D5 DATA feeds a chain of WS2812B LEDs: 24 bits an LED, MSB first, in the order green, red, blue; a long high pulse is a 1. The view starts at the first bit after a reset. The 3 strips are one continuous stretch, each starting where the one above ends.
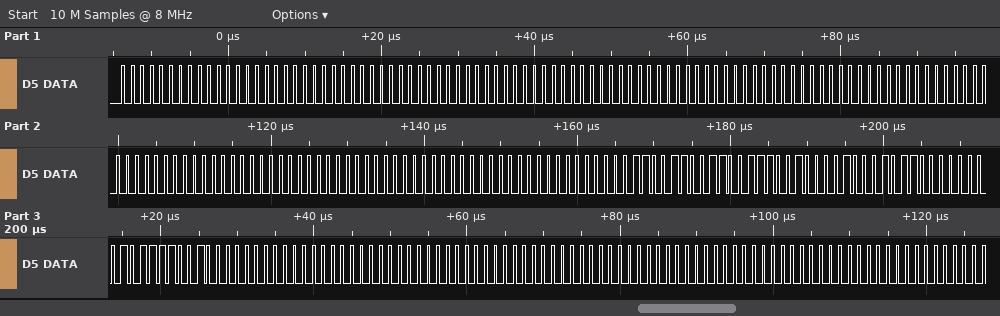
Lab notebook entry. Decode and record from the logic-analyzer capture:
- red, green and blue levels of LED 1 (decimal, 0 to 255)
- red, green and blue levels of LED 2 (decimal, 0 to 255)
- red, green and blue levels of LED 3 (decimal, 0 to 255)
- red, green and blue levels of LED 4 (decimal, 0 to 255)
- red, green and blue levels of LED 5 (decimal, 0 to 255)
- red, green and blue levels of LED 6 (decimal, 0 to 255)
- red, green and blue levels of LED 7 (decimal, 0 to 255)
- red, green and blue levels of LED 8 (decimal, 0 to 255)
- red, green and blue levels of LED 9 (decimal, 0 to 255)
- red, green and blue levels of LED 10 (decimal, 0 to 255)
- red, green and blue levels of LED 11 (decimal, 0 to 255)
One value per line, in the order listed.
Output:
0, 0, 0
0, 0, 0
0, 0, 0
0, 0, 0
0, 0, 0
0, 0, 0
103, 102, 33
1, 22, 121
0, 0, 0
0, 0, 0
0, 0, 0
